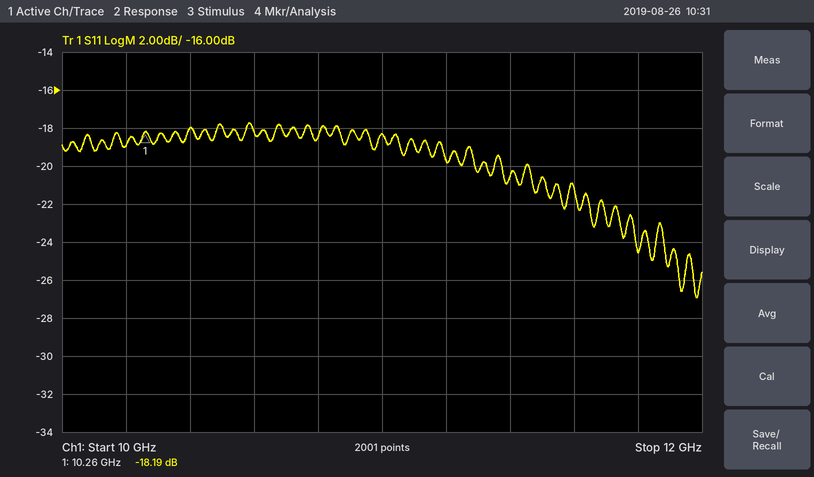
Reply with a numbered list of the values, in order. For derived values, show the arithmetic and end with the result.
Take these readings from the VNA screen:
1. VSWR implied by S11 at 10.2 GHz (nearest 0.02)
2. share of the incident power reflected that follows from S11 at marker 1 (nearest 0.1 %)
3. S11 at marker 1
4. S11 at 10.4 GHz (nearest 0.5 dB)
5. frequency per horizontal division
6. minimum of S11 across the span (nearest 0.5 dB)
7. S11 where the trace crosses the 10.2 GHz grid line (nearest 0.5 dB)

1. |Γ| = 10^(-19/20) = 0.1122; VSWR = (1 + 0.1122)/(1 − 0.1122) ≈ 1.25, so 1.26 to the nearest 0.02
2. 10^(-18.19/10) ≈ 1.5 %
3. -18.19 dB
4. -18.0 dB
5. 200 MHz
6. -27.0 dB
7. -19.0 dB
